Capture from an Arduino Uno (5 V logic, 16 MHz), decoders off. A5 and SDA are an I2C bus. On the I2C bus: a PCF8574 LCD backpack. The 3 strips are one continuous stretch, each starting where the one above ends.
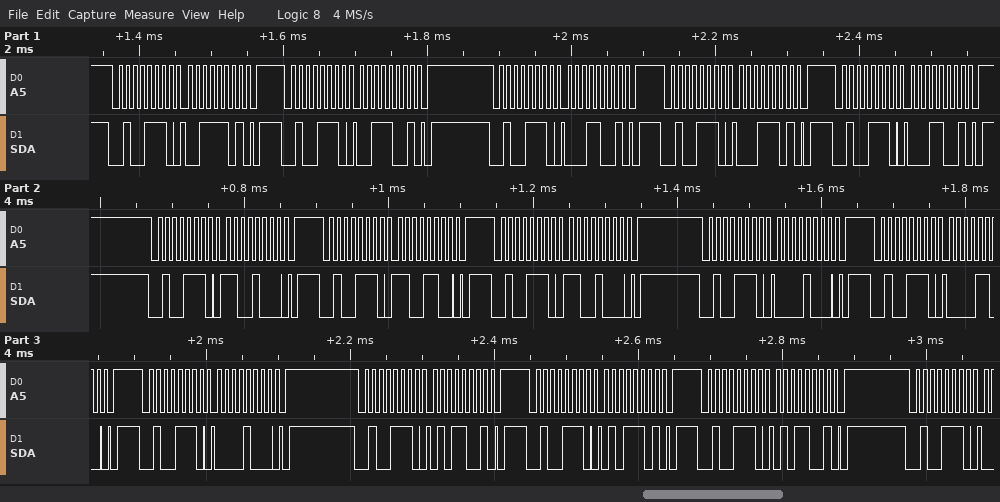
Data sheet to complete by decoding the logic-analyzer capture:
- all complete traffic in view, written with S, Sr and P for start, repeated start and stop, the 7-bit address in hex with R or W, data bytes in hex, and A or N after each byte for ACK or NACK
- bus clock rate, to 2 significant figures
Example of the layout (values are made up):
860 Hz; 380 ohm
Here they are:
S 27W A 3D A P S 27W A 39 A P S 27W A 19 A P S 27W A 1D A P S 27W A 19 A P S 27W A C8 A P S 27W A CC A P S 27W A C8 A P S 27W A 08 A P S 27W A 0C A P S 27W A 08 A P S 27W A 59 A P S 27W A 5D A P S 27W A 59 A P S 27W A; 100 kHz
